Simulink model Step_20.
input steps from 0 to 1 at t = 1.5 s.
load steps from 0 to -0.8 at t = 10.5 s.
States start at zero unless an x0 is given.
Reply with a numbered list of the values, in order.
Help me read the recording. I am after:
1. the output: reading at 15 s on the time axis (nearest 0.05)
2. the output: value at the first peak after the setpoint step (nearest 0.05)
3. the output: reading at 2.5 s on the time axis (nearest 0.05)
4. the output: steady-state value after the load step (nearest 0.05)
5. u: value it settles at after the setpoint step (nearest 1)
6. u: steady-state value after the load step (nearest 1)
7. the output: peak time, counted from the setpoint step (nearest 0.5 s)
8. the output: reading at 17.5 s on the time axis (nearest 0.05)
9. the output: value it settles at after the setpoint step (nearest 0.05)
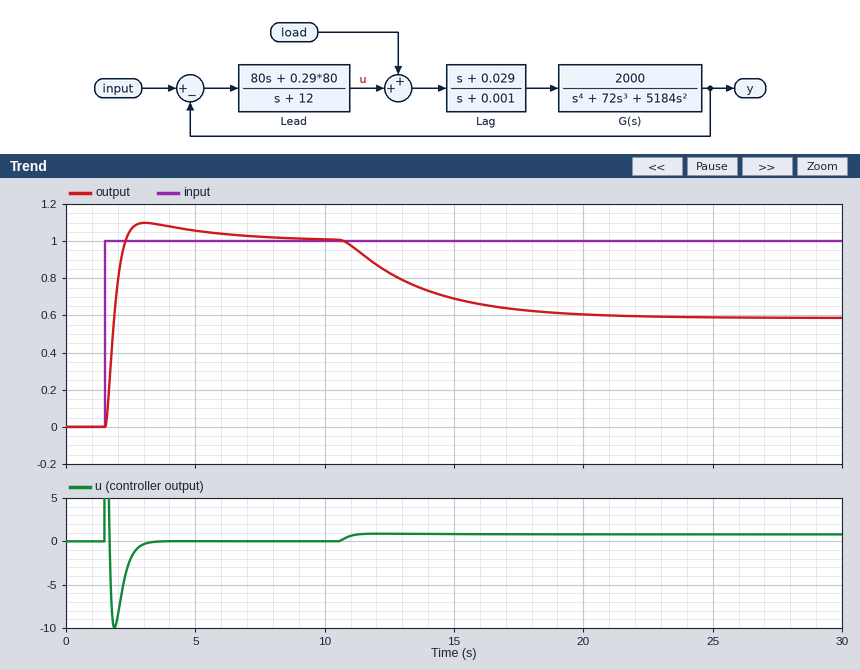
1. 0.70
2. 1.10
3. 1.05
4. 0.60
5. 0
6. 1
7. 1.5 s
8. 0.65
9. 1.00
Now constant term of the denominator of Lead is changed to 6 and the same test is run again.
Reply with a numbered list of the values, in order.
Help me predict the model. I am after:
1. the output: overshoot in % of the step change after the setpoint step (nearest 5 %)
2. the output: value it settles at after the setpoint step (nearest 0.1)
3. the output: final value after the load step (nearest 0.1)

1. 25 %
2. 1.0
3. 0.8
